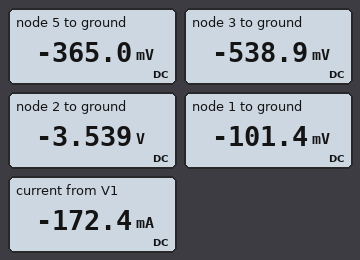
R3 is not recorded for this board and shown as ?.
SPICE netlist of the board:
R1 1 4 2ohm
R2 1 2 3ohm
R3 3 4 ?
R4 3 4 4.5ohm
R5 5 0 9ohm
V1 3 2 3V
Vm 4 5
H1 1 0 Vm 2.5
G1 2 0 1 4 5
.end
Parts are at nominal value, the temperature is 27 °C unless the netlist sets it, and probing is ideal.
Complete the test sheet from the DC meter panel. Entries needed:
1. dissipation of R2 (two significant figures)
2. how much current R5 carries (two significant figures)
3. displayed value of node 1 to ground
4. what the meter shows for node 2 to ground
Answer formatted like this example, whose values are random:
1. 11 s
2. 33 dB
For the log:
1. 3.9 W
2. 41 mA
3. -101.4 mV
4. -3.539 V
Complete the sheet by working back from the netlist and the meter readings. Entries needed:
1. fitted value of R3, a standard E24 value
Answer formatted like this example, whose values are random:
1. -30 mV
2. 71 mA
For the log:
1. 1.3 Ω
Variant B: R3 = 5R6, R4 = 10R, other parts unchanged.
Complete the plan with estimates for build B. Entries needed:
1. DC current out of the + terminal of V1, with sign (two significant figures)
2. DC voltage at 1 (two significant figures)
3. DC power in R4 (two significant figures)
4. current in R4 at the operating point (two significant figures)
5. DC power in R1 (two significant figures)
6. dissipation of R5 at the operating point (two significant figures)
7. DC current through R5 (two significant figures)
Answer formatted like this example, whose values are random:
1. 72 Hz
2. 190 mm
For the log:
1. -200 mA
2. -120 mV
3. 53 mW
4. 73 mA
5. 48 mW
6. 20 mW
7. 48 mA
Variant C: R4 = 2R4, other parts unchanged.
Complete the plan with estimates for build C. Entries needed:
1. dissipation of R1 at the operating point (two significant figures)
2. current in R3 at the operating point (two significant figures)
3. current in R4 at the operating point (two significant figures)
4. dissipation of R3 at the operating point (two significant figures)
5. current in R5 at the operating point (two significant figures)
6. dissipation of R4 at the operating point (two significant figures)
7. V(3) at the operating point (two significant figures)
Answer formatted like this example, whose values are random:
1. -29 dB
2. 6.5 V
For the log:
1. 34 mW
2. 110 mA
3. 60 mA
4. 16 mW
5. 40 mA
6. 8.6 mW
7. -510 mV
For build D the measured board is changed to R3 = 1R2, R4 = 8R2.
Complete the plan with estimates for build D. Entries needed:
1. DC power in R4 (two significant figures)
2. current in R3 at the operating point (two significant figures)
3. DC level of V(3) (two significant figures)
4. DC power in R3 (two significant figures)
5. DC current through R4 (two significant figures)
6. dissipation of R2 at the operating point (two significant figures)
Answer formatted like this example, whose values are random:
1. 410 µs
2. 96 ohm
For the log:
1. 4.0 mW
2. 150 mA
3. -550 mV
4. 27 mW
5. 22 mA
6. 4.0 W
